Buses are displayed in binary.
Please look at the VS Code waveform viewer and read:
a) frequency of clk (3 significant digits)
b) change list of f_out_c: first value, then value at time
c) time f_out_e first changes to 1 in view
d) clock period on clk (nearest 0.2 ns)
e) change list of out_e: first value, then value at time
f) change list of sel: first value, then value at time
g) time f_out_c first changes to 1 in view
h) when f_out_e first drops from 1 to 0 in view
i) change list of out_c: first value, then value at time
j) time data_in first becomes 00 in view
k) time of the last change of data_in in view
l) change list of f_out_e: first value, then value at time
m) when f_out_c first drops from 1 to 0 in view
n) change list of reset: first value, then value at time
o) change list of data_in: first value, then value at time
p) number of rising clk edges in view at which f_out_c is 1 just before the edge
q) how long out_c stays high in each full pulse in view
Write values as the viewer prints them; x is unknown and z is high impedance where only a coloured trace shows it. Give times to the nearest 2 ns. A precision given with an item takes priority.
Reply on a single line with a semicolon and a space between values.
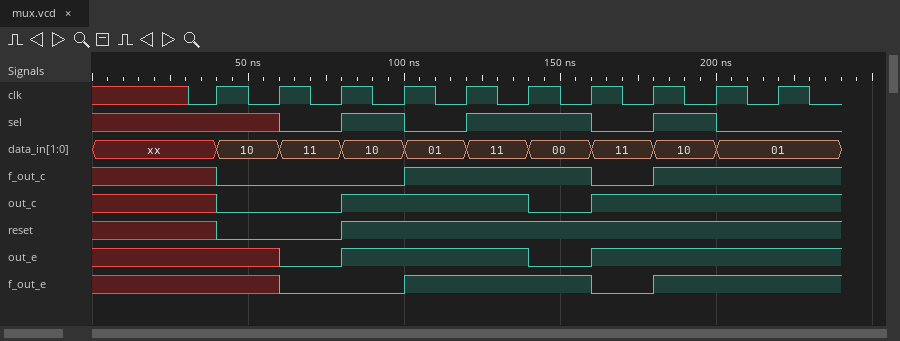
50.0 MHz; x, 0 at 40 ns, 1 at 100 ns, 0 at 160 ns, 1 at 180 ns; 100 ns; 20 ns; x, 0 at 60 ns, 1 at 80 ns, 0 at 140 ns, 1 at 160 ns; x, 0 at 60 ns, 1 at 80 ns, 0 at 100 ns, 1 at 120 ns, 0 at 160 ns, 1 at 180 ns, 0 at 200 ns; 100 ns; 160 ns; x, 0 at 40 ns, 1 at 80 ns, 0 at 140 ns, 1 at 160 ns; 140 ns; 200 ns; x, 0 at 60 ns, 1 at 100 ns, 0 at 160 ns, 1 at 180 ns; 160 ns; x, 0 at 40 ns, 1 at 80 ns; xx, 10 at 40 ns, 11 at 60 ns, 10 at 80 ns, 01 at 100 ns, 11 at 120 ns, 00 at 140 ns, 11 at 160 ns, 10 at 180 ns, 01 at 200 ns; 5; 60 ns
